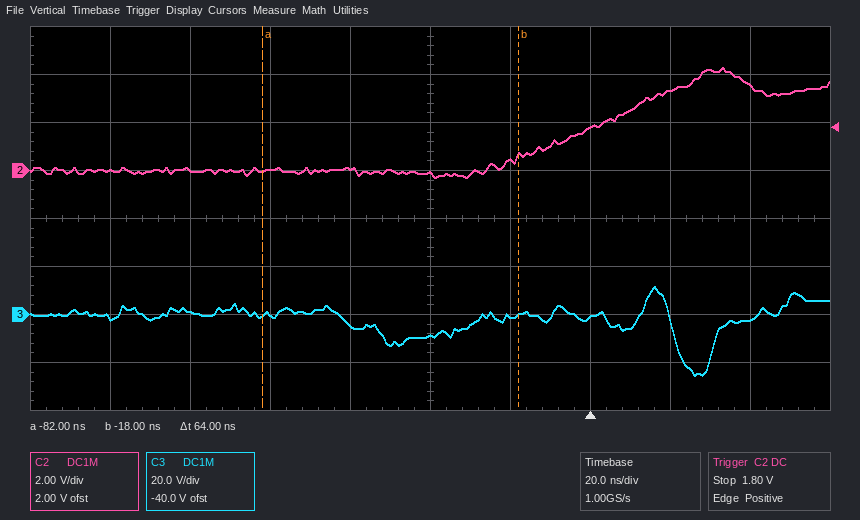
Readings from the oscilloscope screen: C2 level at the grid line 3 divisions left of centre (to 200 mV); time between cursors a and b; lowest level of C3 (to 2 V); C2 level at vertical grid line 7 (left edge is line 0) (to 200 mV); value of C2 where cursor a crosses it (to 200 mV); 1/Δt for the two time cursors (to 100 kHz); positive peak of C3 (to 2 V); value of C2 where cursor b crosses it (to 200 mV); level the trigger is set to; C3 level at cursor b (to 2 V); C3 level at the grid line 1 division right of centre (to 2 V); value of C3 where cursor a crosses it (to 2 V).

0.0 V
64 ns
-26 V
1.8 V
0.0 V
15.6 MHz
12 V
600 mV
1.80 V
0 V
0 V
0 V
